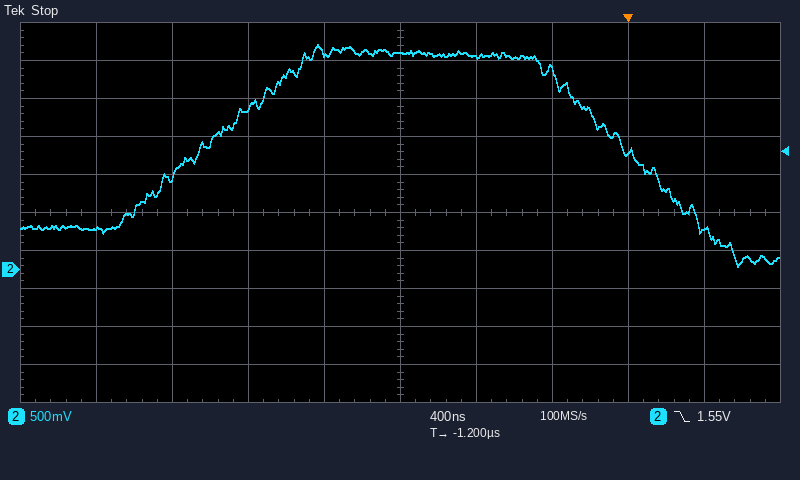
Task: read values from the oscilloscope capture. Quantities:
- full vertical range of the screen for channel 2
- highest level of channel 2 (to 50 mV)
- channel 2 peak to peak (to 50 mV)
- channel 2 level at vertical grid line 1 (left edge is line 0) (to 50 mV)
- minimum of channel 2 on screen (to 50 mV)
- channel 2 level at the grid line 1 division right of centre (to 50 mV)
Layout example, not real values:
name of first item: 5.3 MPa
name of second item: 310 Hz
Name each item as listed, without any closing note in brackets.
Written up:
full vertical range of the screen for channel 2: 5 V
highest level of channel 2: 2.95 V
channel 2 peak to peak: 2.90 V
channel 2 level at vertical grid line 1 (left edge is line 0): 550 mV
minimum of channel 2 on screen: 50 mV
channel 2 level at the grid line 1 division right of centre: 2.80 V
